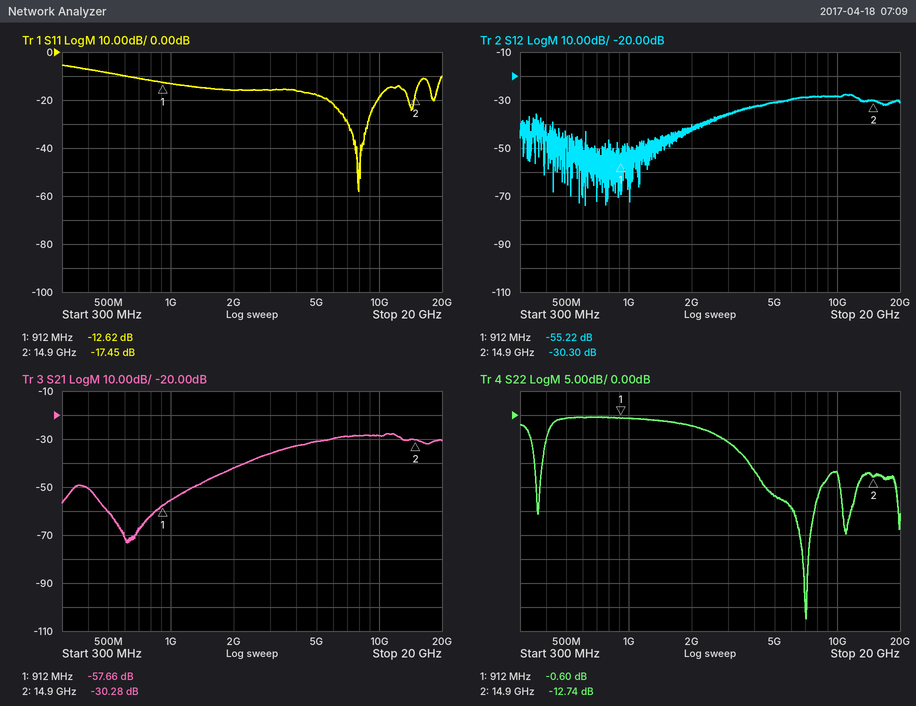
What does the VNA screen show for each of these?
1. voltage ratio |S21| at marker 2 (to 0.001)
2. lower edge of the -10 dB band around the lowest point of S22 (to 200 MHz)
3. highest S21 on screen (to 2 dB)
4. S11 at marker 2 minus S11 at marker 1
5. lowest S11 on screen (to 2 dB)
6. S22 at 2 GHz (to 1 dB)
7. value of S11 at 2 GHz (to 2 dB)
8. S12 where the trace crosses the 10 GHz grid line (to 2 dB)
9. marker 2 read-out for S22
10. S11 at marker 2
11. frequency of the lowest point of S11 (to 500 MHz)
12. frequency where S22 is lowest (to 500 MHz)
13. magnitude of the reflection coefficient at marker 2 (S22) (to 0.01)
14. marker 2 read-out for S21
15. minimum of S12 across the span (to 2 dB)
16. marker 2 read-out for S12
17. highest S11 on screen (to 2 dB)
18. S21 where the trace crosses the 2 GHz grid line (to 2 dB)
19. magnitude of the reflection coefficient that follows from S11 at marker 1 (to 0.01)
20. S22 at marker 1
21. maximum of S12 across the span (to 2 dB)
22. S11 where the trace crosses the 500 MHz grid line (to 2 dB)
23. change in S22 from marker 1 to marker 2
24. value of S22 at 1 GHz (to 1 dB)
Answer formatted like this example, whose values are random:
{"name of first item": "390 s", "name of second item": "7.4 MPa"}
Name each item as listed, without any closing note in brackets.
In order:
{"voltage ratio |S21| at marker 2": "0.031", "lower edge of the -10 dB band around the lowest point of S22": "3.8 GHz", "highest S21 on screen": "-28 dB", "S11 at marker 2 minus S11 at marker 1": "-4.83 dB", "lowest S11 on screen": "-58 dB", "S22 at 2 GHz": "-2 dB", "value of S11 at 2 GHz": "-16 dB", "S12 where the trace crosses the 10 GHz grid line": "-28 dB", "marker 2 read-out for S22": "-12.74 dB", "S11 at marker 2": "-17.45 dB", "frequency of the lowest point of S11": "8.0 GHz", "frequency where S22 is lowest": "7.0 GHz", "magnitude of the reflection coefficient at marker 2 (S22)": "0.23", "marker 2 read-out for S21": "-30.28 dB", "minimum of S12 across the span": "-74 dB", "marker 2 read-out for S12": "-30.30 dB", "highest S11 on screen": "-6 dB", "S21 where the trace crosses the 2 GHz grid line": "-42 dB", "magnitude of the reflection coefficient that follows from S11 at marker 1": "0.23", "S22 at marker 1": "-0.60 dB", "maximum of S12 across the span": "-28 dB", "S11 where the trace crosses the 500 MHz grid line": "-8 dB", "change in S22 from marker 1 to marker 2": "-12.14 dB", "value of S22 at 1 GHz": "-1 dB"}
